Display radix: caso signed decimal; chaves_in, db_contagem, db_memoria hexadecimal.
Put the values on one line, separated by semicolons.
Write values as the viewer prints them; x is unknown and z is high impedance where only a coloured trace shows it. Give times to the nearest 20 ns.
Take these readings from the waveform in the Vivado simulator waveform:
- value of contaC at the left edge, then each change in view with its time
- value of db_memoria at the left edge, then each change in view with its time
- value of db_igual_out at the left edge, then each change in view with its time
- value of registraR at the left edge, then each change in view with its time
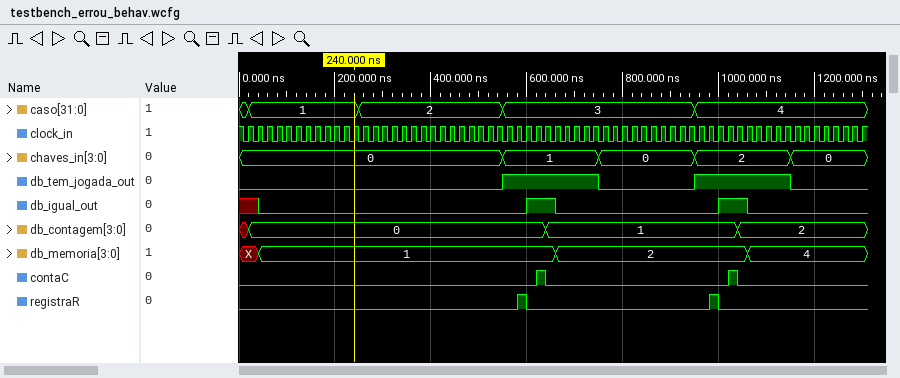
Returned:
0, 1 at 620 ns, 0 at 640 ns, 1 at 1020 ns, 0 at 1040 ns; X, 1 at 40 ns, 2 at 660 ns, 4 at 1060 ns; x, 0 at 40 ns, 1 at 600 ns, 0 at 660 ns, 1 at 1000 ns, 0 at 1060 ns; 0, 1 at 580 ns, 0 at 600 ns, 1 at 980 ns, 0 at 1000 ns
